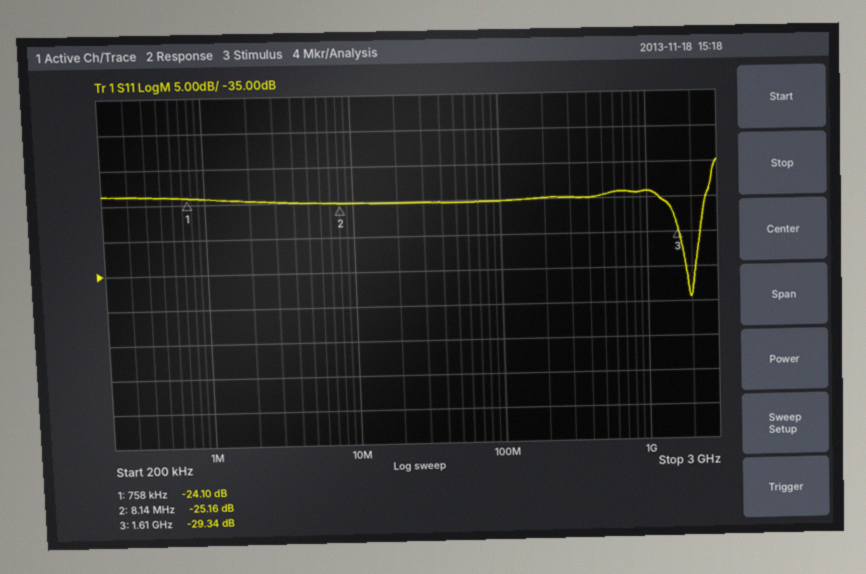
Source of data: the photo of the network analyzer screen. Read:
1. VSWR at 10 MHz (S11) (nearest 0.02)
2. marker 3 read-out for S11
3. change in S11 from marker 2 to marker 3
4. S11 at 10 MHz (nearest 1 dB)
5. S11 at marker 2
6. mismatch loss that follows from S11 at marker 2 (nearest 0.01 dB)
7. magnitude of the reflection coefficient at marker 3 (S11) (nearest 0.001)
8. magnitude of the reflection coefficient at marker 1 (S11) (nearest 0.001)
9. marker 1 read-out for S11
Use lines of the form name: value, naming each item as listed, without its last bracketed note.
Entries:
VSWR at 10 MHz (S11): 1.12
marker 3 read-out for S11: -29.34 dB
change in S11 from marker 2 to marker 3: -4.18 dB
S11 at 10 MHz: -25 dB
S11 at marker 2: -25.16 dB
mismatch loss that follows from S11 at marker 2: 0.01 dB
magnitude of the reflection coefficient at marker 3 (S11): 0.034
magnitude of the reflection coefficient at marker 1 (S11): 0.062
marker 1 read-out for S11: -24.10 dB
